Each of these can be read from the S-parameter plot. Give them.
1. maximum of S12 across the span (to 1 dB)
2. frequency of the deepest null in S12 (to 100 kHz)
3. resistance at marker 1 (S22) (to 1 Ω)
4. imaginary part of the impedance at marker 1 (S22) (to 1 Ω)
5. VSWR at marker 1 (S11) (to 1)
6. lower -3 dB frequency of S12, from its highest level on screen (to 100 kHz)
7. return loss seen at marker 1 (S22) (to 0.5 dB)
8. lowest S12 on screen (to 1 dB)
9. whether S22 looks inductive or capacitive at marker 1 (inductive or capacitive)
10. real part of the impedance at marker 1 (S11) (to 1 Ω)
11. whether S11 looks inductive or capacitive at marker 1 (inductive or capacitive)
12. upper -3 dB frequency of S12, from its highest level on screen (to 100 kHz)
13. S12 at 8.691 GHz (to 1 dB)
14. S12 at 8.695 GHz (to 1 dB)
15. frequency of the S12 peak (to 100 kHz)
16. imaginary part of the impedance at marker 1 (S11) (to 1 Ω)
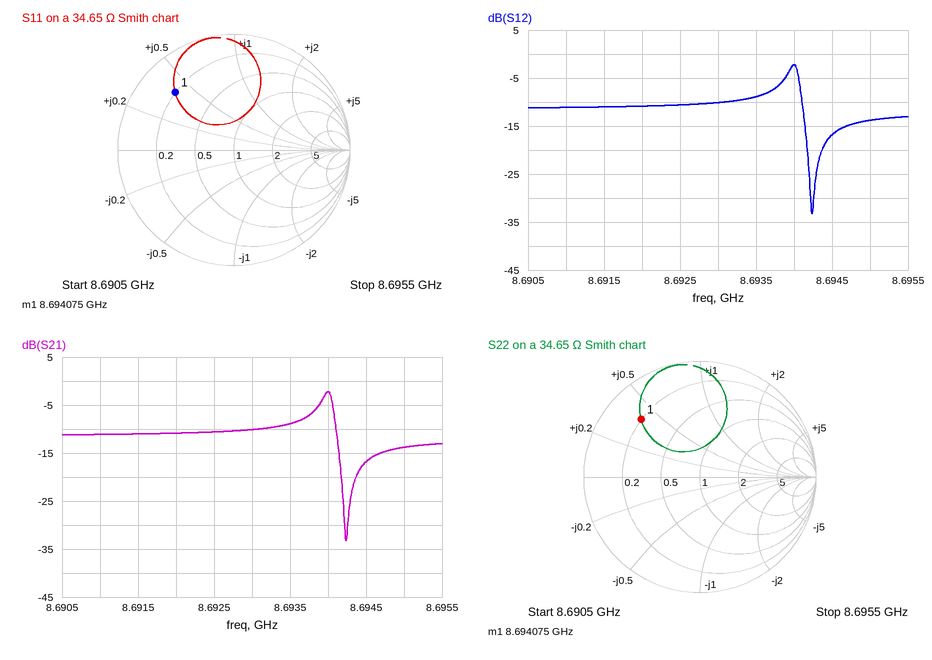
-2 dB
8.6942 GHz
7 Ω
+14 Ω
6
8.6939 GHz
3.0 dB
-33 dB
inductive
7 Ω
inductive
8.6941 GHz
-11 dB
-14 dB
8.6940 GHz
+14 Ω
